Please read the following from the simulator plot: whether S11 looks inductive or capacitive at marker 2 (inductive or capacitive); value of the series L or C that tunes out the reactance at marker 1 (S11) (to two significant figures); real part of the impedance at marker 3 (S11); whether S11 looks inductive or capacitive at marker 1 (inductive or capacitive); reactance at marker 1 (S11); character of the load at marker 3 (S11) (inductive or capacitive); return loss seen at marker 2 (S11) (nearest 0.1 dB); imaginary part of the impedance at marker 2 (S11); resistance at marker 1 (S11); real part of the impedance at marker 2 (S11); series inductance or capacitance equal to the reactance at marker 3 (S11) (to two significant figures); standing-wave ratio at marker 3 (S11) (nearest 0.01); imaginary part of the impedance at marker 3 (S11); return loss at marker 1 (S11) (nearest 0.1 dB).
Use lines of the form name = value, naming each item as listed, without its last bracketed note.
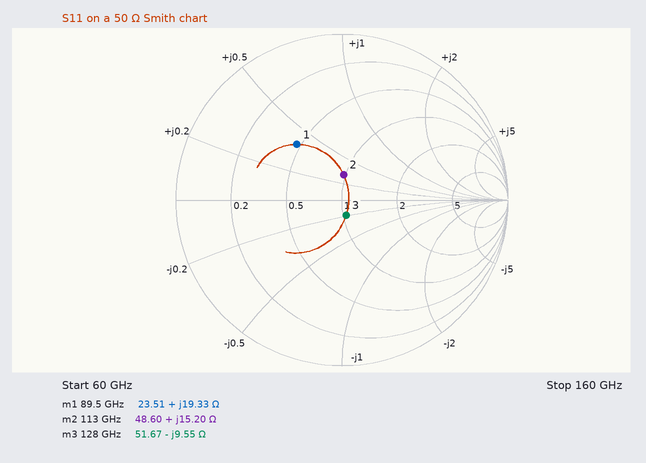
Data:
whether S11 looks inductive or capacitive at marker 2 = inductive
value of the series L or C that tunes out the reactance at marker 1 (S11) = 92 fF
real part of the impedance at marker 3 = 51.67 Ω
whether S11 looks inductive or capacitive at marker 1 = inductive
reactance at marker 1 = +19.33 Ω
character of the load at marker 3 (S11) = capacitive
return loss seen at marker 2 (S11) = 16.3 dB
imaginary part of the impedance at marker 2 = +15.20 Ω
resistance at marker 1 = 23.51 Ω
real part of the impedance at marker 2 = 48.60 Ω
series inductance or capacitance equal to the reactance at marker 3 (S11) = 130 fF
standing-wave ratio at marker 3 (S11) = 1.21
imaginary part of the impedance at marker 3 = -9.55 Ω
return loss at marker 1 (S11) = 7.3 dB
